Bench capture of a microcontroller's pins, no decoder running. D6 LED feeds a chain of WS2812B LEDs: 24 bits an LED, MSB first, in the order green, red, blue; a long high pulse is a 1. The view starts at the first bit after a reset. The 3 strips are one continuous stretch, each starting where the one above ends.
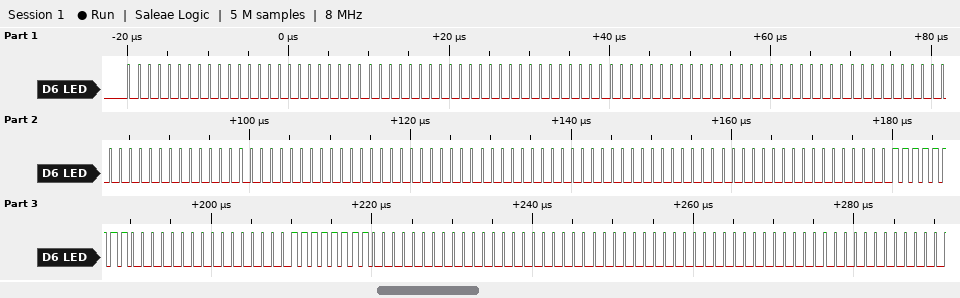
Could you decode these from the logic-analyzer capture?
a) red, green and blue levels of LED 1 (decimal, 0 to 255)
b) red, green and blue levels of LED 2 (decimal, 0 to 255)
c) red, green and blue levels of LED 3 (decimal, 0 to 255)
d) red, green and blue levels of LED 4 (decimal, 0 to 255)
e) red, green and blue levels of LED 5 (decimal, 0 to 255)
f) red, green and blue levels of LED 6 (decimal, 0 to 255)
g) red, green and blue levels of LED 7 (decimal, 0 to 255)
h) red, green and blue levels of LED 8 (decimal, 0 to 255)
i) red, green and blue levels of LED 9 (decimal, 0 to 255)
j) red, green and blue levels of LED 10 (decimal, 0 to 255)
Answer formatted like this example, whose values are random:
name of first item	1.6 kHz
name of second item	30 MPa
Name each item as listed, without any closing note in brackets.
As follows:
red, green and blue levels of LED 1	0, 0, 0
red, green and blue levels of LED 2	0, 0, 0
red, green and blue levels of LED 3	0, 0, 0
red, green and blue levels of LED 4	0, 0, 0
red, green and blue levels of LED 5	0, 0, 0
red, green and blue levels of LED 6	0, 0, 0
red, green and blue levels of LED 7	0, 0, 255
red, green and blue levels of LED 8	0, 0, 255
red, green and blue levels of LED 9	0, 0, 0
red, green and blue levels of LED 10	0, 0, 0
